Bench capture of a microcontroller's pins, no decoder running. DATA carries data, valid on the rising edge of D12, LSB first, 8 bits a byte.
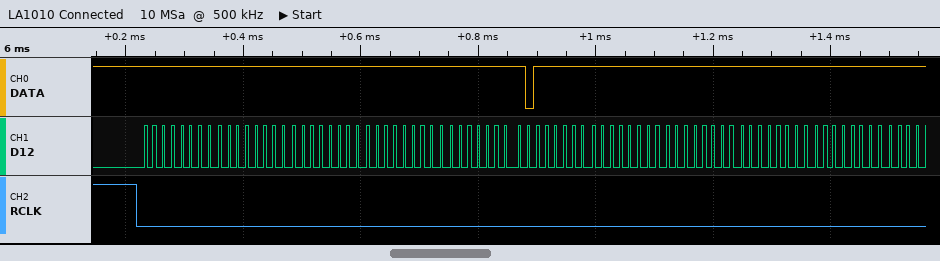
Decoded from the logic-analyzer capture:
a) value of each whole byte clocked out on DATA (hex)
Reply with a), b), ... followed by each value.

a) FF FF FF FF FF FD FF FF FF FF
